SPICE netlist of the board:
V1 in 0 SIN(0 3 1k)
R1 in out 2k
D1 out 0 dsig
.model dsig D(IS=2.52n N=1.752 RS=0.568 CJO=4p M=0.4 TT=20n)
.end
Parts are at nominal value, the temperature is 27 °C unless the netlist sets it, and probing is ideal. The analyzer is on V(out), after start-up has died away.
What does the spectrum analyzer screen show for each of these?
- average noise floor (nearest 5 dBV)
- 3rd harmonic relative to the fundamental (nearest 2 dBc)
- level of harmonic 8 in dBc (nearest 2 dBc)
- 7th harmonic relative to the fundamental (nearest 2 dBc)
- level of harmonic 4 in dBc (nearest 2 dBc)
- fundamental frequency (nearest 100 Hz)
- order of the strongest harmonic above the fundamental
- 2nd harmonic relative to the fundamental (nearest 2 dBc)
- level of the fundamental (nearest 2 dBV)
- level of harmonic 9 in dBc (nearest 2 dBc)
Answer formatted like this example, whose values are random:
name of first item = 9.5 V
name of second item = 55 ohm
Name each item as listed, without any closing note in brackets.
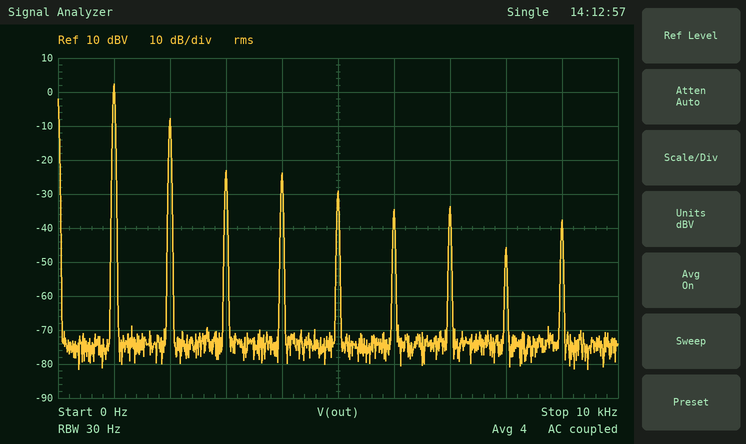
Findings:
average noise floor = -75 dBV
3rd harmonic relative to the fundamental = -26 dBc
level of harmonic 8 in dBc = -48 dBc
7th harmonic relative to the fundamental = -36 dBc
level of harmonic 4 in dBc = -26 dBc
fundamental frequency = 1.0 kHz
order of the strongest harmonic above the fundamental = 2
2nd harmonic relative to the fundamental = -10 dBc
level of the fundamental = 2 dBV
level of harmonic 9 in dBc = -40 dBc
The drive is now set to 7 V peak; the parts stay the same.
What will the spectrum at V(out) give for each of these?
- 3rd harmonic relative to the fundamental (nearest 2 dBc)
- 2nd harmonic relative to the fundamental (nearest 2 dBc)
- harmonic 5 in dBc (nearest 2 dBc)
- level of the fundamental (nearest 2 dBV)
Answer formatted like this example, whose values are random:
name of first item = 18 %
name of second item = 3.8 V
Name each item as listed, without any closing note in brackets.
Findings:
3rd harmonic relative to the fundamental = -30 dBc
2nd harmonic relative to the fundamental = -8 dBc
harmonic 5 in dBc = -36 dBc
level of the fundamental = 8 dBV
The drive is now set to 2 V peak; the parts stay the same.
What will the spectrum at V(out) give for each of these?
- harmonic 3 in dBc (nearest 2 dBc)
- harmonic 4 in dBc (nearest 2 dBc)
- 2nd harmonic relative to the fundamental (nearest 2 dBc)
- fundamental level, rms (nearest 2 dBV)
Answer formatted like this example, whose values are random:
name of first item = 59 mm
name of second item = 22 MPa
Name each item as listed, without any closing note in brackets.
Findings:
harmonic 3 in dBc = -24 dBc
harmonic 4 in dBc = -30 dBc
2nd harmonic relative to the fundamental = -12 dBc
fundamental level, rms = 0 dBV
